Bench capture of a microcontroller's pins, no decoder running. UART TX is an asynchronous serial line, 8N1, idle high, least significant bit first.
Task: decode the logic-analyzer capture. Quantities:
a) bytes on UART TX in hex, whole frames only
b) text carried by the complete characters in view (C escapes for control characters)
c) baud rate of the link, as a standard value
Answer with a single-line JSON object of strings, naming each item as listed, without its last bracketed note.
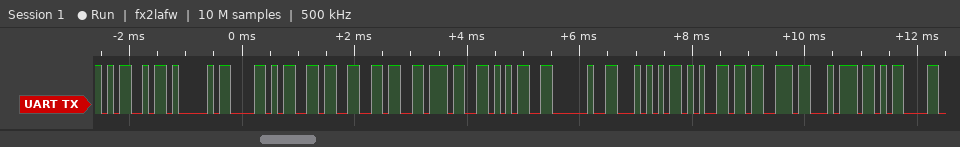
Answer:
{"bytes on UART TX in hex, whole frames only": "4D 41 58 36 36 37 35 20 54 65 73 74 0D", "text carried by the complete characters in view": "\"MAX6675 Test\\r\"", "baud rate of the link, as a standard value": "9600 baud"}
